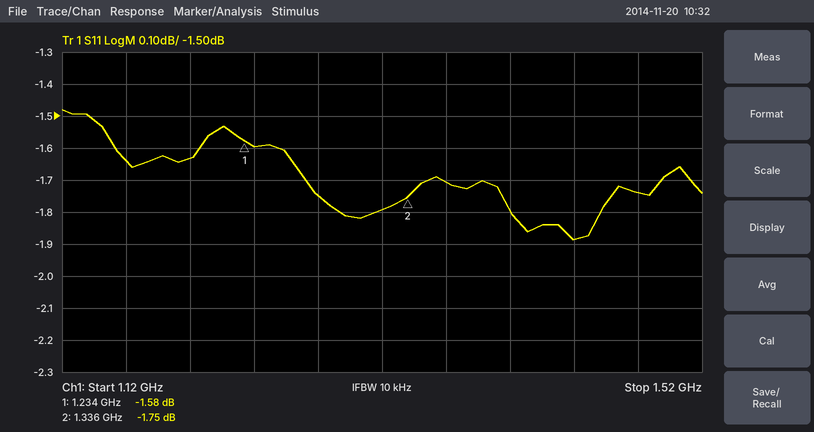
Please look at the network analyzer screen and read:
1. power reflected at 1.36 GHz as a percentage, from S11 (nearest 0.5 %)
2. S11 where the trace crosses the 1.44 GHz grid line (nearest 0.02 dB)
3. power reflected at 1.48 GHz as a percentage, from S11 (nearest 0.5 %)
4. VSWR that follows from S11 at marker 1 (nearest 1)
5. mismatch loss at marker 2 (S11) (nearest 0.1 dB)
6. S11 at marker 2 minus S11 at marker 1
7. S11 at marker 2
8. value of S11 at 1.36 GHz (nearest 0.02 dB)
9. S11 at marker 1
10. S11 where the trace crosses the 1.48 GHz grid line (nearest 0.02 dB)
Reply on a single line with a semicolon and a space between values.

67.5 %; -1.88 dB; 67.0 %; 11; 4.8 dB; -0.17 dB; -1.75 dB; -1.70 dB; -1.58 dB; -1.74 dB
